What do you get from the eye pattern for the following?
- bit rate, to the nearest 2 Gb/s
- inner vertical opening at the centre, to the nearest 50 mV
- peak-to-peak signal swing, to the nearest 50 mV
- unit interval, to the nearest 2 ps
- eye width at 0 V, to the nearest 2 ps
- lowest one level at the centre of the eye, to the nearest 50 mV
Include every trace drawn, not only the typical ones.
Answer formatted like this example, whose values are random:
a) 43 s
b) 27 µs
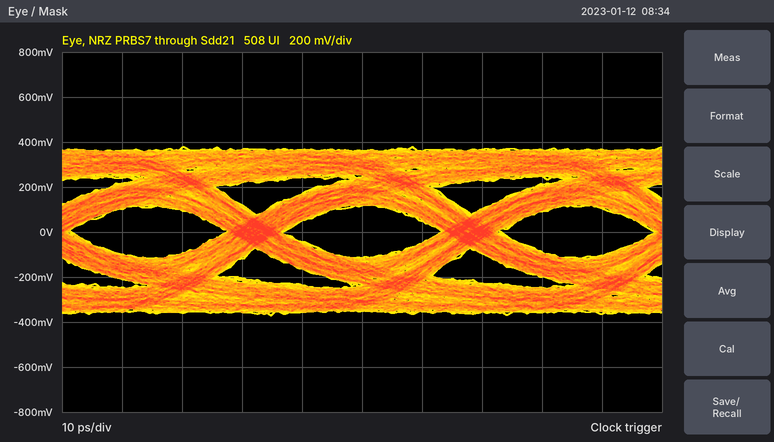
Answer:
a) 28 Gb/s
b) 250 mV
c) 750 mV
d) 36 ps
e) 26 ps
f) 100 mV
